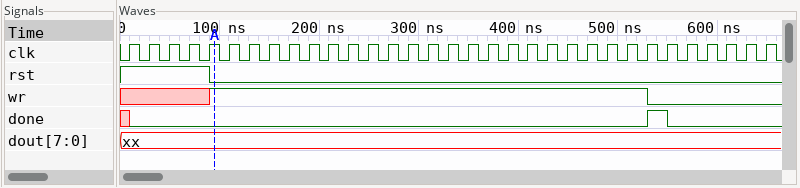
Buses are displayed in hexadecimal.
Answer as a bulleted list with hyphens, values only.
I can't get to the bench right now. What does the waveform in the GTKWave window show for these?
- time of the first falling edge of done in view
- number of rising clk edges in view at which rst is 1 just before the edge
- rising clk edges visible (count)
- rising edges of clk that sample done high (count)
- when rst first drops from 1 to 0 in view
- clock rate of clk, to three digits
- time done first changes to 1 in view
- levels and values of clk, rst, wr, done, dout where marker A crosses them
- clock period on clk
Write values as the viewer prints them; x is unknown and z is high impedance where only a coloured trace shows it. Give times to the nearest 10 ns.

- 550 ns
- 5
- 33
- 1
- 90 ns
- 50.0 MHz
- 530 ns
- clk=1, rst=0, wr=1, done=0, dout=xx
- 20 ns
